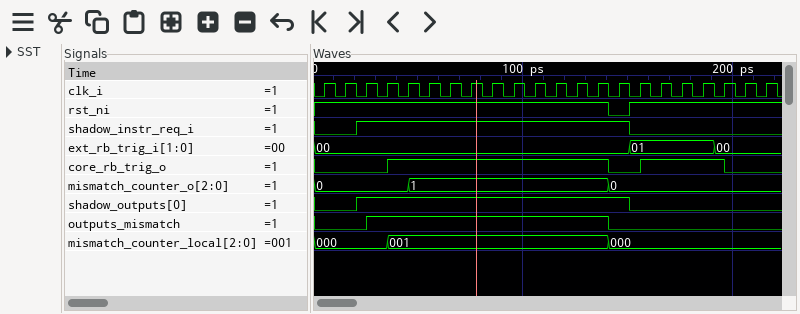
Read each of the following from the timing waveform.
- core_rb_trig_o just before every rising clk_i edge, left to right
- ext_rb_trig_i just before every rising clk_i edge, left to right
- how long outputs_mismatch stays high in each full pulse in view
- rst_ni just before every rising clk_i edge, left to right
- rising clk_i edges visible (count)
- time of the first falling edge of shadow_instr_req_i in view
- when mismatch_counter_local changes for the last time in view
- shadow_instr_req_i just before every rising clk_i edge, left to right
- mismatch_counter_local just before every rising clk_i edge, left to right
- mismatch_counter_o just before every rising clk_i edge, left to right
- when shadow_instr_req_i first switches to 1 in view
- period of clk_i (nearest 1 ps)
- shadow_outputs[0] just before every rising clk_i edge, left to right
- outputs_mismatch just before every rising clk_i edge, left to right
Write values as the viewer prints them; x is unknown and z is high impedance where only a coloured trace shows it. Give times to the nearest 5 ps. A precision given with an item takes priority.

0 0 0 0 1 1 1 1 1 1 1 1 1 1 0 0 1 1 1 1 0 0
00, 00, 00, 00, 00, 00, 00, 00, 00, 00, 00, 00, 00, 00, 00, 01, 01, 01, 01, 00, 00, 00
115 ps
1 1 1 1 1 1 1 1 1 1 1 1 1 1 0 1 1 1 1 1 1 1
22
150 ps
140 ps
0 0 1 1 1 1 1 1 1 1 1 1 1 1 1 0 0 0 0 0 0 0
000, 000, 000, 000, 001, 001, 001, 001, 001, 001, 001, 001, 001, 001, 000, 000, 000, 000, 000, 000, 000, 000
0, 0, 0, 0, 0, 1, 1, 1, 1, 1, 1, 1, 1, 1, 0, 0, 0, 0, 0, 0, 0, 0
20 ps
10 ps
0 0 1 1 1 1 1 1 1 1 1 1 1 1 1 0 0 0 0 0 0 0
0 0 0 1 1 1 1 1 1 1 1 1 1 1 0 0 0 0 0 0 0 0
